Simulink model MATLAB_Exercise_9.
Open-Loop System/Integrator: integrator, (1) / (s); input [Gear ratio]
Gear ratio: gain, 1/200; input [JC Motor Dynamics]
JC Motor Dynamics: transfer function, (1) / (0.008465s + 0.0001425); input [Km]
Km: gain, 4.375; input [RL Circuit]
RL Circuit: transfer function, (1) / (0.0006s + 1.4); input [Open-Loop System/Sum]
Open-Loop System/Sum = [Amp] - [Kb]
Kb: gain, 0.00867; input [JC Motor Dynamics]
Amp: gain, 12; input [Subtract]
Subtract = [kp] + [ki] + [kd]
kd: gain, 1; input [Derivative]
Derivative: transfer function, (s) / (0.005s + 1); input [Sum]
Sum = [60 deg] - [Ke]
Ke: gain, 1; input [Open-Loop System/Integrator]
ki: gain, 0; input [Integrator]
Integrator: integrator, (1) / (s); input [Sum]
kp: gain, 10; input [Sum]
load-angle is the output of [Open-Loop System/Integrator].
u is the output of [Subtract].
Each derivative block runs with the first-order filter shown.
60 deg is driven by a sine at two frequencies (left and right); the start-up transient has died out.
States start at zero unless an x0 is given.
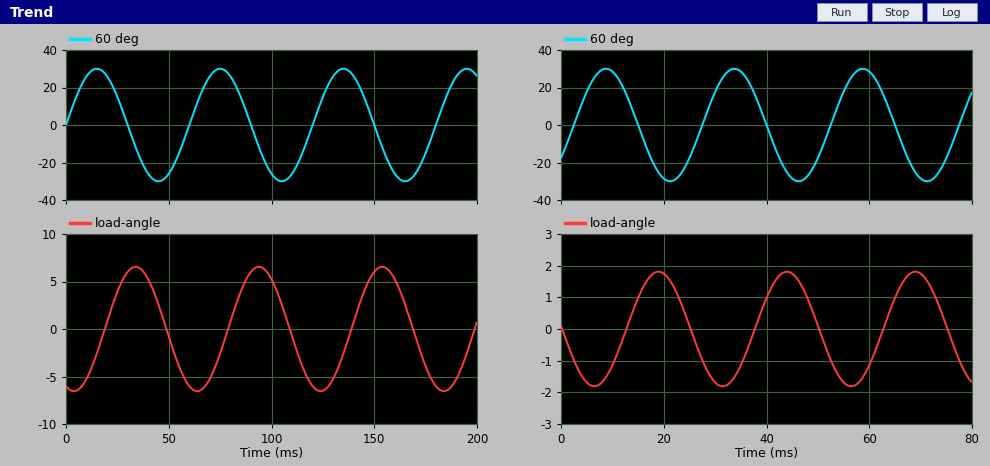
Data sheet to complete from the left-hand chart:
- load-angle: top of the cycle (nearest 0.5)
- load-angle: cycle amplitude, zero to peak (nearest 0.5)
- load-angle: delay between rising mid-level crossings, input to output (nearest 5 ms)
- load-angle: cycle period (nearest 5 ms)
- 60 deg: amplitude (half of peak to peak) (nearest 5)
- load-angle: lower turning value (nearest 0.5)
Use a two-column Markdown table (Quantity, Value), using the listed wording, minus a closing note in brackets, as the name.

| Quantity | Value |
|---|---|
| load-angle: top of the cycle | 6.5 |
| load-angle: cycle amplitude, zero to peak | 6.5 |
| load-angle: delay between rising mid-level crossings, input to output | 20 ms |
| load-angle: cycle period | 60 ms |
| 60 deg: amplitude (half of peak to peak) | 30 |
| load-angle: lower turning value | -6.5 |
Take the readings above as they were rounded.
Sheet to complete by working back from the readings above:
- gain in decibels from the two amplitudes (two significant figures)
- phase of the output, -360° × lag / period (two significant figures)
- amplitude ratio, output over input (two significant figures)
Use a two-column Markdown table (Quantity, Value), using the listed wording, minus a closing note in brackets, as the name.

| Quantity | Value |
|---|---|
| gain in decibels from the two amplitudes | -13 dB |
| phase of the output, -360° × lag / period | -120° |
| amplitude ratio, output over input | 0.22 |
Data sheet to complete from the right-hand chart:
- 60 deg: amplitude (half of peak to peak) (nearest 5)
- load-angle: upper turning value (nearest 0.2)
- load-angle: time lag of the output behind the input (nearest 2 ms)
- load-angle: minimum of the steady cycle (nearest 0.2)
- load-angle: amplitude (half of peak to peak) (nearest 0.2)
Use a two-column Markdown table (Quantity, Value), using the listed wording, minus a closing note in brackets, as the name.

| Quantity | Value |
|---|---|
| 60 deg: amplitude (half of peak to peak) | 30 |
| load-angle: upper turning value | 1.8 |
| load-angle: time lag of the output behind the input | 10 ms |
| load-angle: minimum of the steady cycle | -1.8 |
| load-angle: amplitude (half of peak to peak) | 1.8 |
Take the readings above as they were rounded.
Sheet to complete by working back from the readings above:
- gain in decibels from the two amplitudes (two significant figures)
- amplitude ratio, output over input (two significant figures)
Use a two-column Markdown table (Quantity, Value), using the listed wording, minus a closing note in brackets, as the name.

| Quantity | Value |
|---|---|
| gain in decibels from the two amplitudes | -24 dB |
| amplitude ratio, output over input | 0.060 |
